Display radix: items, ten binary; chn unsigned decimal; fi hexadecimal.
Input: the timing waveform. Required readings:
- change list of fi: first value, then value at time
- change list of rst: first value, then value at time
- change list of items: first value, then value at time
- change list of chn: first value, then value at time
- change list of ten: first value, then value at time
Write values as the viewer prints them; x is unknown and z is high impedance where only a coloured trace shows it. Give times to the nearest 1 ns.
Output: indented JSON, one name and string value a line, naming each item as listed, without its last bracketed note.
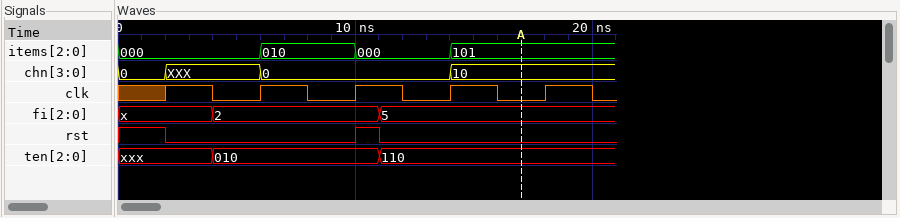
{
  "change list of fi: first value, then value at time": "x, 2 at 4 ns, 5 at 11 ns",
  "change list of rst: first value, then value at time": "1, 0 at 2 ns, 1 at 10 ns, 0 at 11 ns",
  "change list of items: first value, then value at time": "000, 010 at 6 ns, 000 at 10 ns, 101 at 14 ns",
  "change list of chn: first value, then value at time": "0, XXX at 2 ns, 0 at 6 ns, 10 at 14 ns",
  "change list of ten: first value, then value at time": "xxx, 010 at 4 ns, 110 at 11 ns"
}
